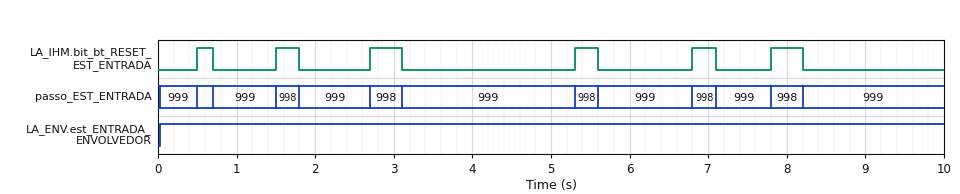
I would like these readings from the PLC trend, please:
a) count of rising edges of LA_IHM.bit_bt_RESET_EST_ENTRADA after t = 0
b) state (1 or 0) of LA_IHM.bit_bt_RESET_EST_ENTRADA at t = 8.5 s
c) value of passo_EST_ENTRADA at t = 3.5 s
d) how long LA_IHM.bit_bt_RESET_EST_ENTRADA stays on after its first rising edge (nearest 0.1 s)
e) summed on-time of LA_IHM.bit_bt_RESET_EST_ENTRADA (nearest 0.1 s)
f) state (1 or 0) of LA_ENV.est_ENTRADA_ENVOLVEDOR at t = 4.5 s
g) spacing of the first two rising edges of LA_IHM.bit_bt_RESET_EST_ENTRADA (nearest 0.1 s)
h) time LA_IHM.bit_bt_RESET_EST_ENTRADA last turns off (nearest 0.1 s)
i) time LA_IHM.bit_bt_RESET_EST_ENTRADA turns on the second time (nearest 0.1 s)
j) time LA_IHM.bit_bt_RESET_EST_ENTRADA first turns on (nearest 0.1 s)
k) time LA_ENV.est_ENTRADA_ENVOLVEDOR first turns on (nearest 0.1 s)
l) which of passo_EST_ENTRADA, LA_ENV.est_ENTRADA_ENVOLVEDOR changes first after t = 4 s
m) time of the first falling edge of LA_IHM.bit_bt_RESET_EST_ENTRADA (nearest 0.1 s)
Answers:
6
0
999
0.2 s
1.9 s
1
1.0 s
8.2 s
1.5 s
0.5 s
0.0 s
passo_EST_ENTRADA
0.7 s
